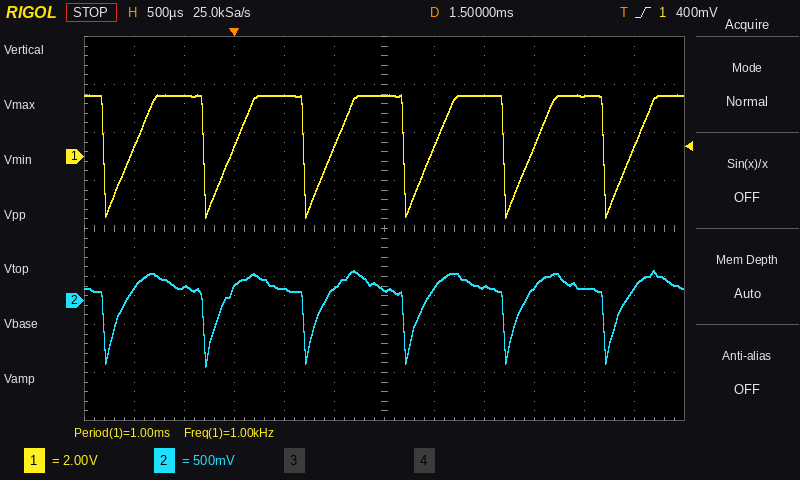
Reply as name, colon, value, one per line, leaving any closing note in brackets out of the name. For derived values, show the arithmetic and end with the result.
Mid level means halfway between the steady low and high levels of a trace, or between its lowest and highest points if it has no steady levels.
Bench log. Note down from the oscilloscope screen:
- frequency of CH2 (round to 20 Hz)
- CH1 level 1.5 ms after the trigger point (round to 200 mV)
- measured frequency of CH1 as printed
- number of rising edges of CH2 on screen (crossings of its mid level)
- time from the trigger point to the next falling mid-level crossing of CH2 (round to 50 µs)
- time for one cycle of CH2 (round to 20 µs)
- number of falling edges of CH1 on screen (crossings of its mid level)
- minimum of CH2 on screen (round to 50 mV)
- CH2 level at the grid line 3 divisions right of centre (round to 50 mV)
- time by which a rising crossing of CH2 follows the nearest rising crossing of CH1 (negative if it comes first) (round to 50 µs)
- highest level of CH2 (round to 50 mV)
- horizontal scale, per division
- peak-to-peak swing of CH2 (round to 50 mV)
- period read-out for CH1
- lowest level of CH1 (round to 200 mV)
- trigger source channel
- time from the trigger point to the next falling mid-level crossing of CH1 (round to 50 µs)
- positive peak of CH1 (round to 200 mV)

frequency of CH2: 1 / 1.00 ms ≈ 1.00 kHz
CH1 level 1.5 ms after the trigger point: 2.6 V
measured frequency of CH1 as printed: 1.00 kHz
number of rising edges of CH2 on screen: 6
time from the trigger point to the next falling mid-level crossing of CH2: 700 µs
time for one cycle of CH2: 1.00 ms
number of falling edges of CH1 on screen: 6
minimum of CH2 on screen: -700 mV
CH2 level at the grid line 3 divisions right of centre: 150 mV
time by which a rising crossing of CH2 follows the nearest rising crossing of CH1 (negative if it comes first): -150 µs
highest level of CH2: 300 mV
horizontal scale, per division: 500 µs
peak-to-peak swing of CH2: 300 mV − (-700 mV) = 1.00 V
period read-out for CH1: 1.00 ms
lowest level of CH1: -2.6 V
trigger source channel: CH1
time from the trigger point to the next falling mid-level crossing of CH1: 700 µs
positive peak of CH1: 2.6 V
